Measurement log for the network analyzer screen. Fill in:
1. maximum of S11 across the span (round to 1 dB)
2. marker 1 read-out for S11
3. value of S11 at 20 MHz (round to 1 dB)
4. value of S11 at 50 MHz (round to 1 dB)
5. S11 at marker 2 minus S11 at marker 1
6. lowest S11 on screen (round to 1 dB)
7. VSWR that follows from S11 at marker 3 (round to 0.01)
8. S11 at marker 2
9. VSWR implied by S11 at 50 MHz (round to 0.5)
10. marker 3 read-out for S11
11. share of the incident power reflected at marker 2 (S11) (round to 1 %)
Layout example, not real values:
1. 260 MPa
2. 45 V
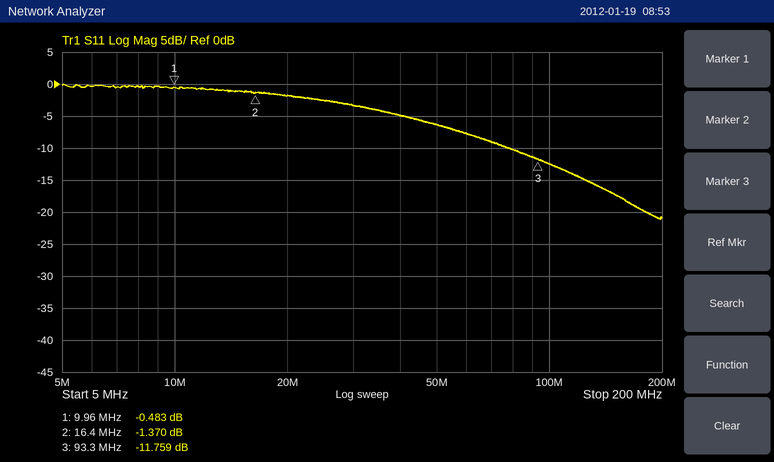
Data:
1. 0 dB
2. -0.483 dB
3. -2 dB
4. -6 dB
5. -0.887 dB
6. -21 dB
7. 1.70
8. -1.370 dB
9. 3.0
10. -11.759 dB
11. 73 %
